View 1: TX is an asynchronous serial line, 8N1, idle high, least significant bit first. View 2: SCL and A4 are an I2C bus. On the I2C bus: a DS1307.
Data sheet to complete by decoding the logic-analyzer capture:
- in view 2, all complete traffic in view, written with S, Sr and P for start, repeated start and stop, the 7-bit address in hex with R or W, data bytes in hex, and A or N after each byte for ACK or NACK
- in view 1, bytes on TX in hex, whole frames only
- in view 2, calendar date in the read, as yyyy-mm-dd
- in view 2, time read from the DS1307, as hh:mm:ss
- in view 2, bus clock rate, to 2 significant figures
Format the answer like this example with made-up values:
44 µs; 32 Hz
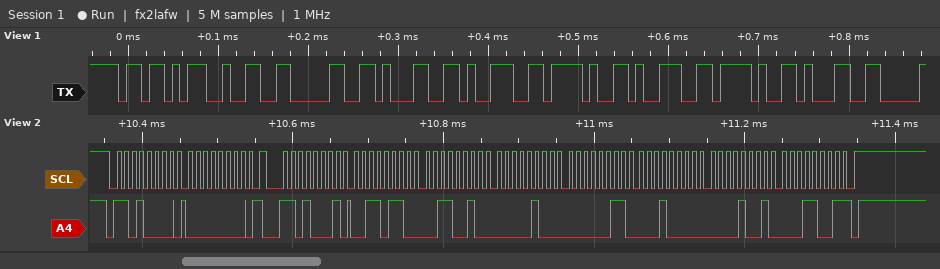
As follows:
S 68W A 00 A Sr 68R A 36 A 32 A 04 A 03 A 10 A 09 A 19 N P; 5B 32 30 31 39 2F 39 2F 31; 2019-09-10; 04:32:36; 100 kHz
